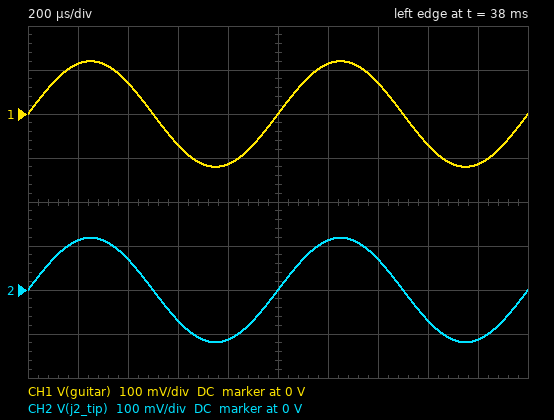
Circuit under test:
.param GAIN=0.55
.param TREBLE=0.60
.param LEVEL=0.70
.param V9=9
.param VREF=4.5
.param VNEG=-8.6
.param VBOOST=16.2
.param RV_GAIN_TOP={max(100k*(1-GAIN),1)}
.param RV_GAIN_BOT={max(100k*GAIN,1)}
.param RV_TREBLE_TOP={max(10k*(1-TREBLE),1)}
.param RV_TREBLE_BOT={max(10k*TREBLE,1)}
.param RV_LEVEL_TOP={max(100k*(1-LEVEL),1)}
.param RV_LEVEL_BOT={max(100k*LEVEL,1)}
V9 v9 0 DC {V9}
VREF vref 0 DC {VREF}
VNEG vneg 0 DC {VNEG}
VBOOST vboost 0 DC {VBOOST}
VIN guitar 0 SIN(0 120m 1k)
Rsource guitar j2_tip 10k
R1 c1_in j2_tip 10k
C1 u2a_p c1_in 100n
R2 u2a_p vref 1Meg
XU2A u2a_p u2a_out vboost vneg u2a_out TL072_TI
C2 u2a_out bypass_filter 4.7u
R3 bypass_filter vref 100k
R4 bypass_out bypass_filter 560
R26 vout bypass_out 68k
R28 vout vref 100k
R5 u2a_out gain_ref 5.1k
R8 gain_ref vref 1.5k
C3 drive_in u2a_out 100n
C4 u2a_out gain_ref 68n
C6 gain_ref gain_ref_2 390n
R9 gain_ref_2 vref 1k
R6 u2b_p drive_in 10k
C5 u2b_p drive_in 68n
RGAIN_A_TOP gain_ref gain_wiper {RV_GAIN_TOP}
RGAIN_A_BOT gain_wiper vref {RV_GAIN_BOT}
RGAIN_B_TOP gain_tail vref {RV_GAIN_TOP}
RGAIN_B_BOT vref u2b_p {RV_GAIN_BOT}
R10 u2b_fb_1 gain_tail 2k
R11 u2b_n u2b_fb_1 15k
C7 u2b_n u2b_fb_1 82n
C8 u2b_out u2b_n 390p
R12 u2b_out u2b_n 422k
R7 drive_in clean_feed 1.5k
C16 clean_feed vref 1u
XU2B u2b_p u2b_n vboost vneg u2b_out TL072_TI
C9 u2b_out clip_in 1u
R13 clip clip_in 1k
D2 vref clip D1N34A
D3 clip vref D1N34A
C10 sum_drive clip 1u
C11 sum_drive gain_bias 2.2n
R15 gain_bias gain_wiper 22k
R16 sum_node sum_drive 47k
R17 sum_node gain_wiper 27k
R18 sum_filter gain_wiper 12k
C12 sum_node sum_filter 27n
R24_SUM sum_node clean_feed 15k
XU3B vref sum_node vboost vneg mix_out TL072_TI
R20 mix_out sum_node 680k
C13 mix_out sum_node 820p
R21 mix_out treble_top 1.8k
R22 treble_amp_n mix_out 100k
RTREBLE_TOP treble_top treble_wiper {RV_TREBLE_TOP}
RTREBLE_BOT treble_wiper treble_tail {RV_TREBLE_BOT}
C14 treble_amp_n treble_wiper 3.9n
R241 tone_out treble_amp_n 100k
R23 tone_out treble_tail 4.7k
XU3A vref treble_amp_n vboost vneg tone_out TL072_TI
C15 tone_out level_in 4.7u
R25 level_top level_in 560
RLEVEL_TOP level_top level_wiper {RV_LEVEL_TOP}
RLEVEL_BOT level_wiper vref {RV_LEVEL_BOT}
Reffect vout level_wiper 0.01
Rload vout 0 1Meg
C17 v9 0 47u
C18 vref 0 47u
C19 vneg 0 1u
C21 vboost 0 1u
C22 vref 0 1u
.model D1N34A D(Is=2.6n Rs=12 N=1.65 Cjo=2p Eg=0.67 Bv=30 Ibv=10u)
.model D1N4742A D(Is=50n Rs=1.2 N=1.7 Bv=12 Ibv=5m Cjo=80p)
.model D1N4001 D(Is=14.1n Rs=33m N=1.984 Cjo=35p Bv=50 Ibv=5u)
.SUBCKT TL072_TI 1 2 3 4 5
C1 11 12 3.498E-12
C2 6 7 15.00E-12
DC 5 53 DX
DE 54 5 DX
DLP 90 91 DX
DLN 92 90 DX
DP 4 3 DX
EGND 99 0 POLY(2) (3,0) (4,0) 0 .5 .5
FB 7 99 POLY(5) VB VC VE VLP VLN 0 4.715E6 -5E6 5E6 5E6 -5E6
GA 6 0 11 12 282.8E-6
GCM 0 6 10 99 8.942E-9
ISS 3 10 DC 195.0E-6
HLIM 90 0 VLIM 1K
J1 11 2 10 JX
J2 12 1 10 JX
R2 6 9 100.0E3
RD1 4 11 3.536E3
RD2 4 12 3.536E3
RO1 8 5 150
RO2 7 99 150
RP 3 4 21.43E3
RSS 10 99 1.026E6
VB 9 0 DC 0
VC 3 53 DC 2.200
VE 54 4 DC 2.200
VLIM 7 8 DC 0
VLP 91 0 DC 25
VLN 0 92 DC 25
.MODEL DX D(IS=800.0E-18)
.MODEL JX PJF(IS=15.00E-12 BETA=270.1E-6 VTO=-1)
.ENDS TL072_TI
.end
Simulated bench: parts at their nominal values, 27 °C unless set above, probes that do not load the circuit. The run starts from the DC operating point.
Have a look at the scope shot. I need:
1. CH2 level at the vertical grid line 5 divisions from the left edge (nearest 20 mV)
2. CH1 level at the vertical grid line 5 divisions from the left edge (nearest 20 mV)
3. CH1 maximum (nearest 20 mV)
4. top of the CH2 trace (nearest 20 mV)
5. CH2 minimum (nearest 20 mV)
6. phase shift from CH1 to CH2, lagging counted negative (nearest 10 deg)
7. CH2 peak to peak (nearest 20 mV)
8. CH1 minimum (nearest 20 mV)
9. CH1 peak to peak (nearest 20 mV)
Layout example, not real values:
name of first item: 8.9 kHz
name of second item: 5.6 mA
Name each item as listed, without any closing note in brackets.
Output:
CH2 level at the vertical grid line 5 divisions from the left edge: 0 V
CH1 level at the vertical grid line 5 divisions from the left edge: 0 V
CH1 maximum: 120 mV
top of the CH2 trace: 120 mV
CH2 minimum: -120 mV
phase shift from CH1 to CH2, lagging counted negative: 0 deg
CH2 peak to peak: 240 mV
CH1 minimum: -120 mV
CH1 peak to peak: 240 mV
